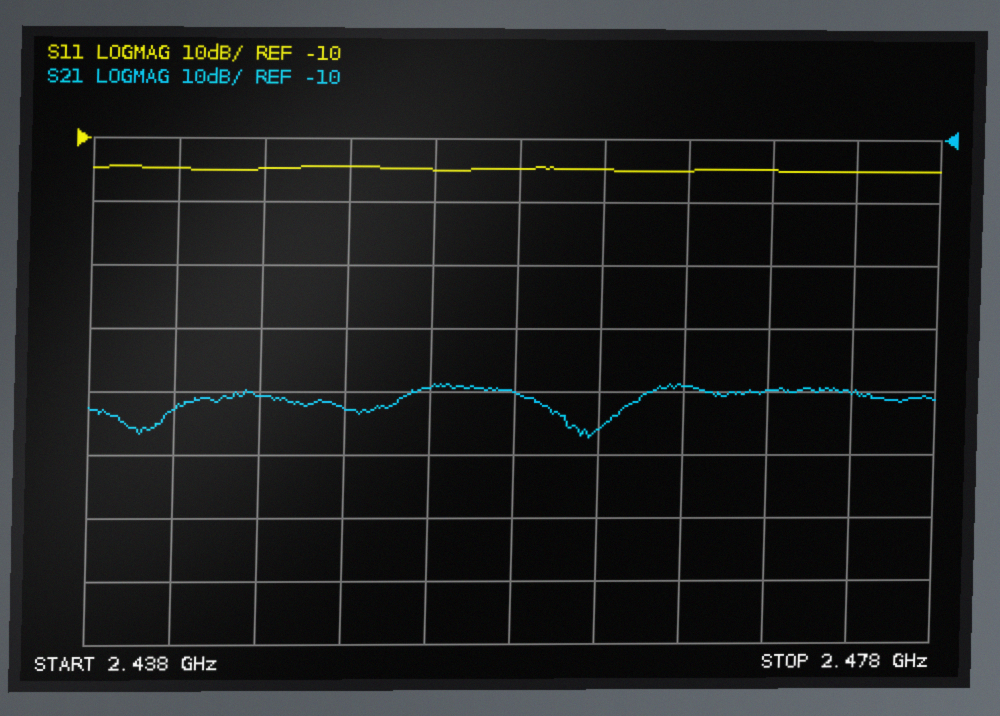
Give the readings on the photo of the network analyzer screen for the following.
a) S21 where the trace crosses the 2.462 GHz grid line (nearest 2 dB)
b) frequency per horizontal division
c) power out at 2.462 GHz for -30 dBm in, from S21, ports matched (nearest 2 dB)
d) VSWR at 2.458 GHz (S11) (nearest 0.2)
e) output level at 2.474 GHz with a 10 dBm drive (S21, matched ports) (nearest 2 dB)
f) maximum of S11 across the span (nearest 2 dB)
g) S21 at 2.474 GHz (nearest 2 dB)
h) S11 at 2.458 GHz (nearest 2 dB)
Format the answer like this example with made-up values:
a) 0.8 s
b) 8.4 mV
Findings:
a) -56 dB
b) 4 MHz
c) -86 dBm
d) 1.4
e) -40 dBm
f) -14 dB
g) -50 dB
h) -14 dB
